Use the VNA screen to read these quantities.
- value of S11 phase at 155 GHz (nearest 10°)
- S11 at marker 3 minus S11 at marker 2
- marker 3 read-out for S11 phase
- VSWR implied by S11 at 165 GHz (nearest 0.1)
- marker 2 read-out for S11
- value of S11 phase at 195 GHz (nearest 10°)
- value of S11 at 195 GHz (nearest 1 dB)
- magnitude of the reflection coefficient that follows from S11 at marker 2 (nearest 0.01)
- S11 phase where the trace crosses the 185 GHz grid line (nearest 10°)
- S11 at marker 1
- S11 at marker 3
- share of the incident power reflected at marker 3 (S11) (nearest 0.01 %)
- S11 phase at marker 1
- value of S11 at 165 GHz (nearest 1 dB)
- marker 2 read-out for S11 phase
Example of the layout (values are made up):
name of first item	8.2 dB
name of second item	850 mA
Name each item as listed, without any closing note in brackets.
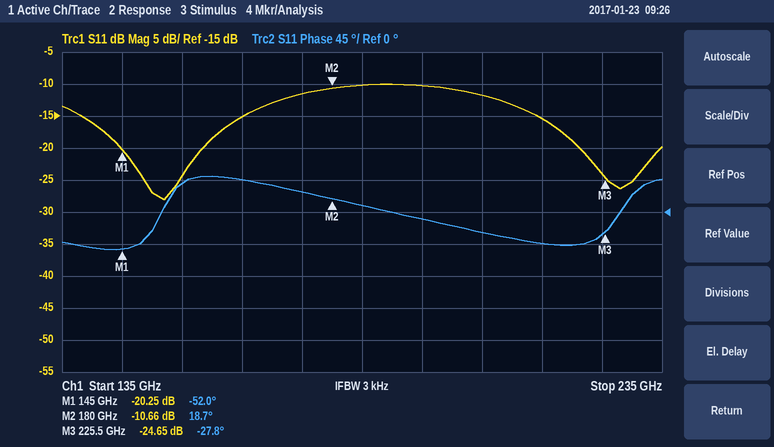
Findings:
value of S11 phase at 155 GHz	40°
S11 at marker 3 minus S11 at marker 2	-13.99 dB
marker 3 read-out for S11 phase	-27.8°
VSWR implied by S11 at 165 GHz	1.4
marker 2 read-out for S11	-10.66 dB
value of S11 phase at 195 GHz	-10°
value of S11 at 195 GHz	-10 dB
magnitude of the reflection coefficient that follows from S11 at marker 2	0.29
S11 phase where the trace crosses the 185 GHz grid line	10°
S11 at marker 1	-20.25 dB
S11 at marker 3	-24.65 dB
share of the incident power reflected at marker 3 (S11)	0.34 %
S11 phase at marker 1	-52.0°
value of S11 at 165 GHz	-15 dB
marker 2 read-out for S11 phase	18.7°
